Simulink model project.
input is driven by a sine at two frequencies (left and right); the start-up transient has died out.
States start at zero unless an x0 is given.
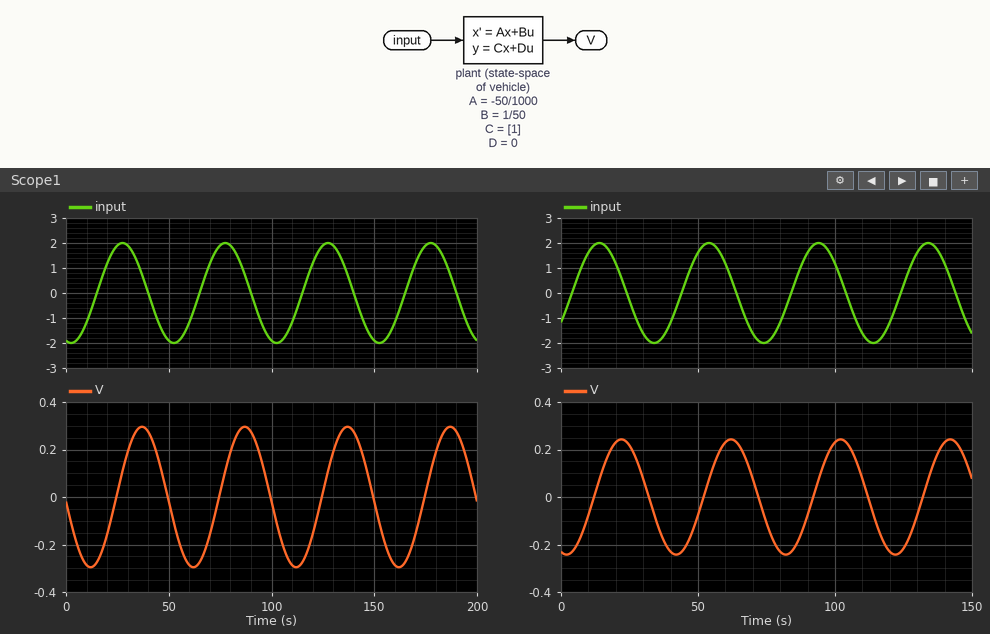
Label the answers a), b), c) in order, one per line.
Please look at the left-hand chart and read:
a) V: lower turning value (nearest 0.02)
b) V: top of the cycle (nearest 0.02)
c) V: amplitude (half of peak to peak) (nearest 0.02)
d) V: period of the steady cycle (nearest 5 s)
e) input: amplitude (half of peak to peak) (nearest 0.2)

a) -0.30
b) 0.30
c) 0.30
d) 50 s
e) 2.0
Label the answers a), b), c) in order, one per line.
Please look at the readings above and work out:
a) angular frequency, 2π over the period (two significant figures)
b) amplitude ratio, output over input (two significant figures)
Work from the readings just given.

a) 0.13 rad/s
b) 0.15
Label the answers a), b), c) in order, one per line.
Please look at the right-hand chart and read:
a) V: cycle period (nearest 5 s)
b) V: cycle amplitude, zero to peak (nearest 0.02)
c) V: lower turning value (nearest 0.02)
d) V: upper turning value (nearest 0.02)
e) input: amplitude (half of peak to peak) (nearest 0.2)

a) 40 s
b) 0.24
c) -0.24
d) 0.24
e) 2.0
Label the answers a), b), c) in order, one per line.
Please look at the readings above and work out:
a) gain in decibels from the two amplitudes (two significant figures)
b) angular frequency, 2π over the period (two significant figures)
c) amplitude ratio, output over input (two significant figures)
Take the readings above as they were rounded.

a) -18 dB
b) 0.16 rad/s
c) 0.12
